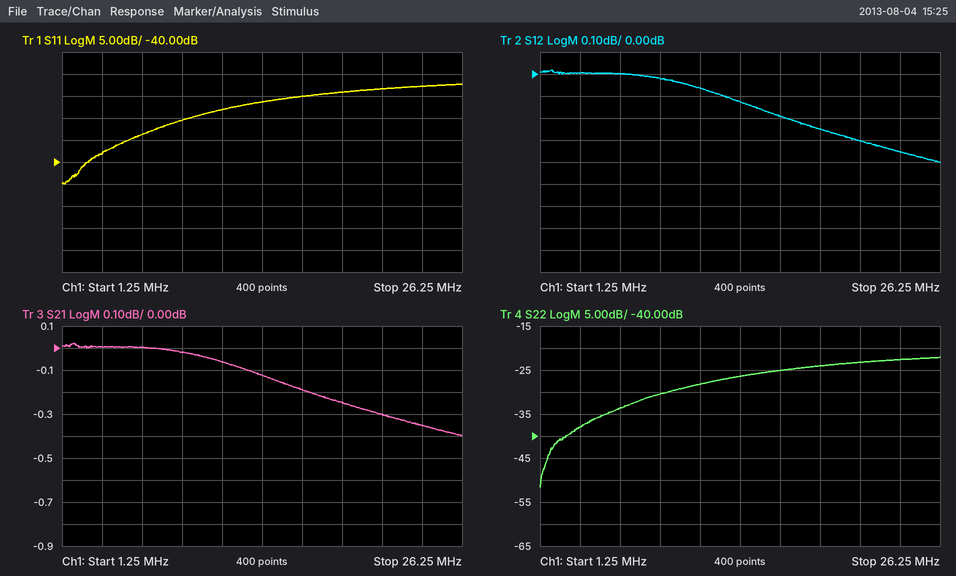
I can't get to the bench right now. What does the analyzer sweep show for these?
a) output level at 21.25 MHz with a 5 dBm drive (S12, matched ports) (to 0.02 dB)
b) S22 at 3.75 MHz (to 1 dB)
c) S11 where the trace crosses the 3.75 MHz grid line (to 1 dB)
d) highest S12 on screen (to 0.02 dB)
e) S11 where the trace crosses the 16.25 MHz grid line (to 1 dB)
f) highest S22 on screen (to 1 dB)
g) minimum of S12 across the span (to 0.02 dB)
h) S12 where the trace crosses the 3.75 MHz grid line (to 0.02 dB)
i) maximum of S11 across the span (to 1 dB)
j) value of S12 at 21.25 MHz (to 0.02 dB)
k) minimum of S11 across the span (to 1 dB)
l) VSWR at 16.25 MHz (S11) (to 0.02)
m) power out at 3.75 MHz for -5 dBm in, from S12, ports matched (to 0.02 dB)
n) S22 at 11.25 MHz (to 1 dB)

4.70 dBm
-38 dB
-38 dB
0.02 dB
-25 dB
-22 dB
-0.40 dB
0.00 dB
-22 dB
-0.30 dB
-45 dB
1.12
-5.00 dBm
-28 dB
